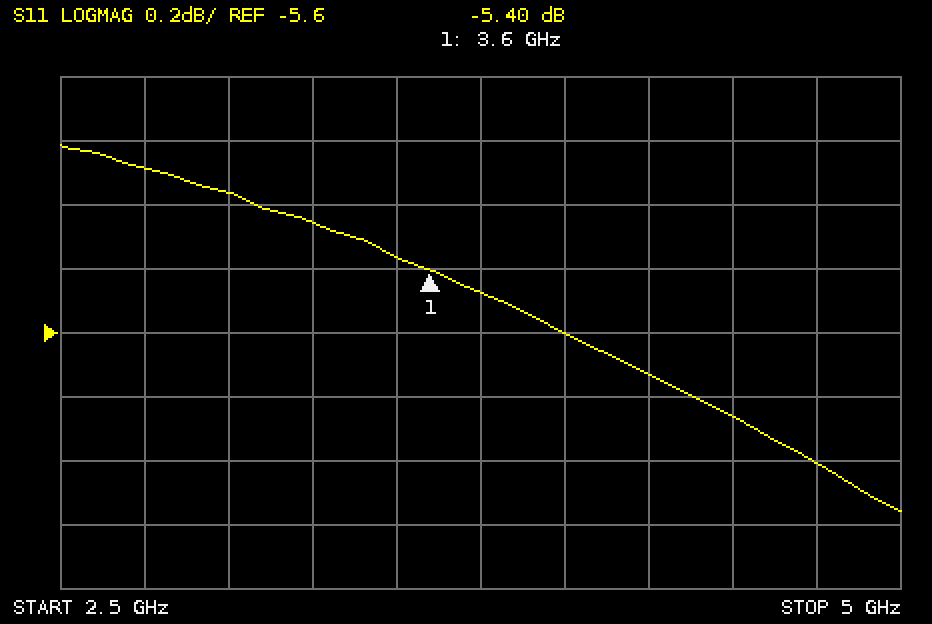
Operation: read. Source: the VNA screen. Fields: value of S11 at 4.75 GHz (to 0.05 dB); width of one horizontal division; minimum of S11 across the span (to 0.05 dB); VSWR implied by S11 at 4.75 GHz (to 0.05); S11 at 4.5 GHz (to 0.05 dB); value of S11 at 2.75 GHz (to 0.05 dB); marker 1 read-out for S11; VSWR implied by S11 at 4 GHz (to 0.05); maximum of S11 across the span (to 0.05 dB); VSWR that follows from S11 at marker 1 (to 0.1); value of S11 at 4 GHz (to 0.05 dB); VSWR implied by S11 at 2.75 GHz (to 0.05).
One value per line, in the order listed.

-6.00 dB
250 MHz
-6.15 dB
3.00
-5.85 dB
-5.10 dB
-5.40 dB
3.20
-5.00 dB
3.3
-5.60 dB
3.50
